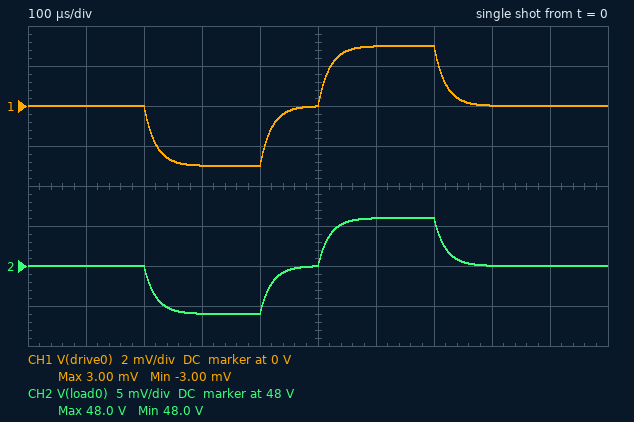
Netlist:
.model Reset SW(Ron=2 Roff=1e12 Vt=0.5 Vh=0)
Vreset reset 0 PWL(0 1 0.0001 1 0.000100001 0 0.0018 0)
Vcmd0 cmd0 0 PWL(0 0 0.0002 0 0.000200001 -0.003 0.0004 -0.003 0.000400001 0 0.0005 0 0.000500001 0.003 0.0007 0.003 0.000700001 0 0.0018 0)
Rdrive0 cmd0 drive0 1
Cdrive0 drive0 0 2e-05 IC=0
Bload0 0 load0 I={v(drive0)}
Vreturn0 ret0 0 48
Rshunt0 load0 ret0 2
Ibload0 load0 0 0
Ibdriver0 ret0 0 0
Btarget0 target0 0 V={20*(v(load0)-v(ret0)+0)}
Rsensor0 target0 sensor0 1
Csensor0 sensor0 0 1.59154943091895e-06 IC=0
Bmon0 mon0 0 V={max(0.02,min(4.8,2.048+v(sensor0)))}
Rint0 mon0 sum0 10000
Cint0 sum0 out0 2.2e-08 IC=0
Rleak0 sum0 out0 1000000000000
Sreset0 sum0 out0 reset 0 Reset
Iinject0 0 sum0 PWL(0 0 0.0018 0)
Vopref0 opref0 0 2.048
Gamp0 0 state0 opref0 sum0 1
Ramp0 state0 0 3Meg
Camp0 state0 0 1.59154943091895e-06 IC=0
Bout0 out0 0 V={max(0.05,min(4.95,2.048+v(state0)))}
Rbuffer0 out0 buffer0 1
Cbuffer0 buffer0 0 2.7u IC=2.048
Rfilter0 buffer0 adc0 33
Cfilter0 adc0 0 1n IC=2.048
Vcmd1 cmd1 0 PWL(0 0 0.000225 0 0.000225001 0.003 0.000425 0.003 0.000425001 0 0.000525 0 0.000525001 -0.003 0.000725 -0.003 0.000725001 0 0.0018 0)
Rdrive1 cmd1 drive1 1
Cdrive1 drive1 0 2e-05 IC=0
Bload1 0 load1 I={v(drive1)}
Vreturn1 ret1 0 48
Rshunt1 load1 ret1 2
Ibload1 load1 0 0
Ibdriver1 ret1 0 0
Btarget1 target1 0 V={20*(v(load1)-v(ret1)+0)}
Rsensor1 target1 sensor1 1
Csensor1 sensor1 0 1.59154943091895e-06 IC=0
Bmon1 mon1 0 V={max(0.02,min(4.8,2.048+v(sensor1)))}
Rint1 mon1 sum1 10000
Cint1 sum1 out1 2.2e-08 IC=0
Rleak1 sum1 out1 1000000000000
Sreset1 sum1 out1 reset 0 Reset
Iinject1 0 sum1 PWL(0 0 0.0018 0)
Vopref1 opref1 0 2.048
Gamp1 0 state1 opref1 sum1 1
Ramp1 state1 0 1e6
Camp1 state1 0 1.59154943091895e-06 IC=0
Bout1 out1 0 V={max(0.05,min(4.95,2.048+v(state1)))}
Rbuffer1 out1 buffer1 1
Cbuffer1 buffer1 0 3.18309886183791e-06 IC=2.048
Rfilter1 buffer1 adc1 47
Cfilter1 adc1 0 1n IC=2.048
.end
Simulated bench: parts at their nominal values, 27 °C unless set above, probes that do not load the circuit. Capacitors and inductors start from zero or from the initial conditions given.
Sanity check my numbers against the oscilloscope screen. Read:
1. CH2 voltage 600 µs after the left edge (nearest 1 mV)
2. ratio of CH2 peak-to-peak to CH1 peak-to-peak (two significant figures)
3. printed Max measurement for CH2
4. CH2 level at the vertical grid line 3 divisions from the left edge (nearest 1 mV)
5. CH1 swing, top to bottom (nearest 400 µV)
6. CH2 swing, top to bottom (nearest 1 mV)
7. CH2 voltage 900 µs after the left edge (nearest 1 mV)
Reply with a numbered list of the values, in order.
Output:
1. 48.006 V
2. 2.0
3. 48.0 V
4. 47.994 V
5. 6.0 mV
6. 12 mV
7. 48.000 V
